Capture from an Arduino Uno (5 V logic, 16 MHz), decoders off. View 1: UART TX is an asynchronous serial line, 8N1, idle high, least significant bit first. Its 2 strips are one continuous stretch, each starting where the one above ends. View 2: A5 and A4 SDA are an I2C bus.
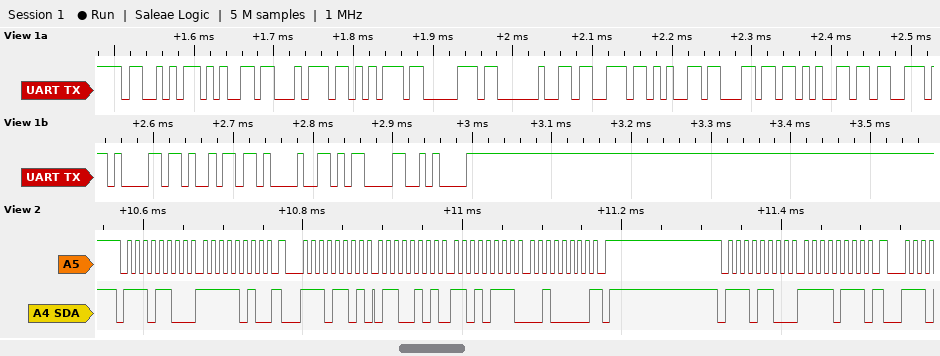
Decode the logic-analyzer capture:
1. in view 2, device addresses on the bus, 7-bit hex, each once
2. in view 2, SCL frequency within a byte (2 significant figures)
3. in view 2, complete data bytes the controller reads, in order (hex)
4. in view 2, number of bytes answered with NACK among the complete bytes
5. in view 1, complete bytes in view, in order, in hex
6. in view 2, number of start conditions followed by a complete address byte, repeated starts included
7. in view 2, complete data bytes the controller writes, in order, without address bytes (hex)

0x76
100 kHz
65 D7 20
1
0x53 0x65 0x74 0x75 0x70 0x20 0x73 0x65 0x6C 0x65 0x73 0x61 0x69 0x21 0x0D 0x0A
3
FA F7
